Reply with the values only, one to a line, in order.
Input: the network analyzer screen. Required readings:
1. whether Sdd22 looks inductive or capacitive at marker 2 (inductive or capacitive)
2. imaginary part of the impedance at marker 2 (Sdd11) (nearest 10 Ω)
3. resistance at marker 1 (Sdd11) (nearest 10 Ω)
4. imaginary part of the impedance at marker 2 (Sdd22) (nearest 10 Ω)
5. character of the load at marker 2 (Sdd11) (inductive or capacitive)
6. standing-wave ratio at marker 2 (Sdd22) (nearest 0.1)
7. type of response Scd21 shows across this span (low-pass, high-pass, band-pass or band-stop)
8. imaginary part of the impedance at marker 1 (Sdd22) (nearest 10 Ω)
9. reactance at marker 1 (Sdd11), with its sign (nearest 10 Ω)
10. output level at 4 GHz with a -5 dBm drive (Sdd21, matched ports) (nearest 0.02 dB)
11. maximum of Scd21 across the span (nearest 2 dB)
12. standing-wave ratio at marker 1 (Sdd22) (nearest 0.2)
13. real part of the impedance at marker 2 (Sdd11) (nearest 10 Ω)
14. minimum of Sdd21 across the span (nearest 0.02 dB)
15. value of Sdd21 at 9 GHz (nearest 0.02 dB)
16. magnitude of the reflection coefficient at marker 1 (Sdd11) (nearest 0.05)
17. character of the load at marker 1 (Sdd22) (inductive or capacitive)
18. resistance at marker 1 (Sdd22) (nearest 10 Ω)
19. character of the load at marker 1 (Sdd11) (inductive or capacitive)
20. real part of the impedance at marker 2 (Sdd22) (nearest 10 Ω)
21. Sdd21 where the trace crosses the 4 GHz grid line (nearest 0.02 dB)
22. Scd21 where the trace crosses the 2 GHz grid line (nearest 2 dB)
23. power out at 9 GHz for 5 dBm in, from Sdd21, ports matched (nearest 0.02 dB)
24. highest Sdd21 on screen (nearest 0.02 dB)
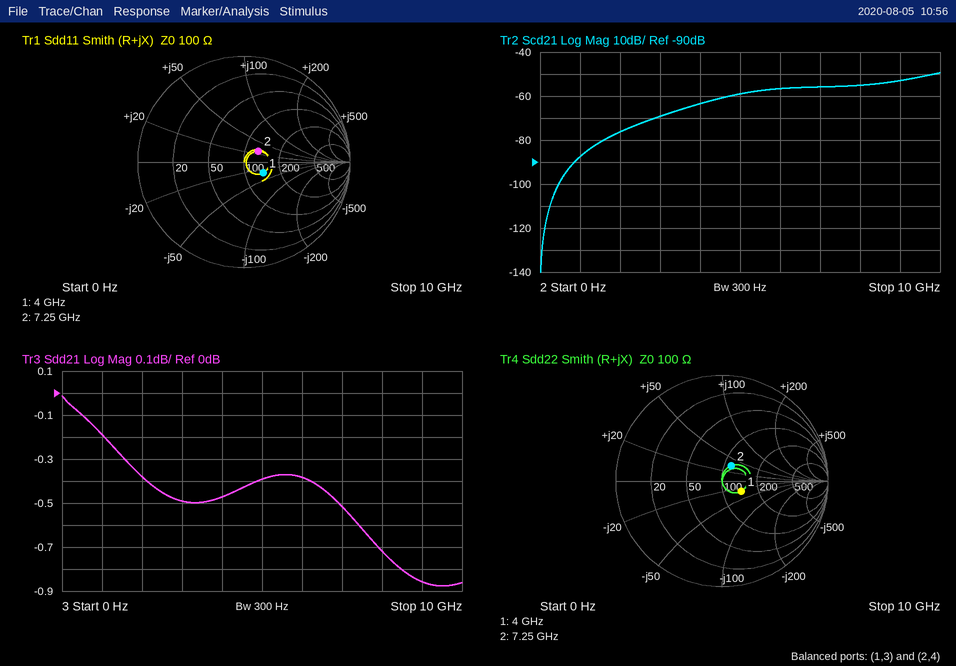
inductive
+30 Ω
140 Ω
+30 Ω
inductive
1.4
high-pass
-30 Ω
-30 Ω
-5.48 dBm
-50 dB
1.6
130 Ω
-0.88 dB
-0.86 dB
0.20
capacitive
140 Ω
capacitive
110 Ω
-0.48 dB
-76 dB
4.14 dBm
-0.02 dB
